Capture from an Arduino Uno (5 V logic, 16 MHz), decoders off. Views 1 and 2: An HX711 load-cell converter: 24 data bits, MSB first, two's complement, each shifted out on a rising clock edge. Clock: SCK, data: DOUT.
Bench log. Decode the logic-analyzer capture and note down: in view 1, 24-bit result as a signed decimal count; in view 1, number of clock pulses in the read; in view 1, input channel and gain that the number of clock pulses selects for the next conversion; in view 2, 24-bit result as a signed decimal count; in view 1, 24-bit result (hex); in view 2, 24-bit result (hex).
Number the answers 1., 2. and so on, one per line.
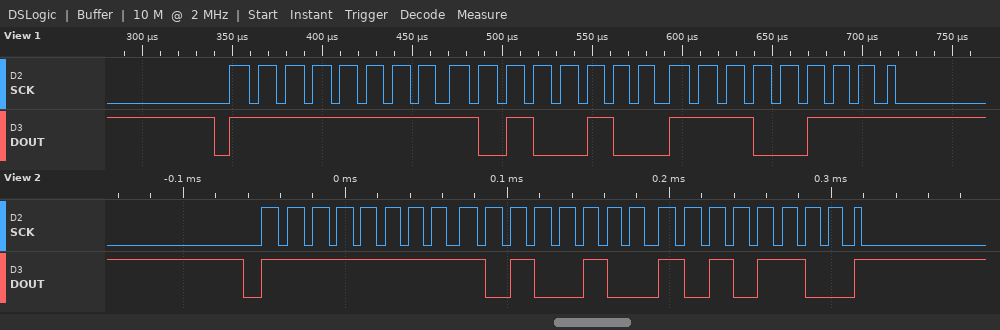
1. -23321
2. 25
3. channel A, gain 128
4. -23380
5. 0xFFA4E7
6. 0xFFA4AC
